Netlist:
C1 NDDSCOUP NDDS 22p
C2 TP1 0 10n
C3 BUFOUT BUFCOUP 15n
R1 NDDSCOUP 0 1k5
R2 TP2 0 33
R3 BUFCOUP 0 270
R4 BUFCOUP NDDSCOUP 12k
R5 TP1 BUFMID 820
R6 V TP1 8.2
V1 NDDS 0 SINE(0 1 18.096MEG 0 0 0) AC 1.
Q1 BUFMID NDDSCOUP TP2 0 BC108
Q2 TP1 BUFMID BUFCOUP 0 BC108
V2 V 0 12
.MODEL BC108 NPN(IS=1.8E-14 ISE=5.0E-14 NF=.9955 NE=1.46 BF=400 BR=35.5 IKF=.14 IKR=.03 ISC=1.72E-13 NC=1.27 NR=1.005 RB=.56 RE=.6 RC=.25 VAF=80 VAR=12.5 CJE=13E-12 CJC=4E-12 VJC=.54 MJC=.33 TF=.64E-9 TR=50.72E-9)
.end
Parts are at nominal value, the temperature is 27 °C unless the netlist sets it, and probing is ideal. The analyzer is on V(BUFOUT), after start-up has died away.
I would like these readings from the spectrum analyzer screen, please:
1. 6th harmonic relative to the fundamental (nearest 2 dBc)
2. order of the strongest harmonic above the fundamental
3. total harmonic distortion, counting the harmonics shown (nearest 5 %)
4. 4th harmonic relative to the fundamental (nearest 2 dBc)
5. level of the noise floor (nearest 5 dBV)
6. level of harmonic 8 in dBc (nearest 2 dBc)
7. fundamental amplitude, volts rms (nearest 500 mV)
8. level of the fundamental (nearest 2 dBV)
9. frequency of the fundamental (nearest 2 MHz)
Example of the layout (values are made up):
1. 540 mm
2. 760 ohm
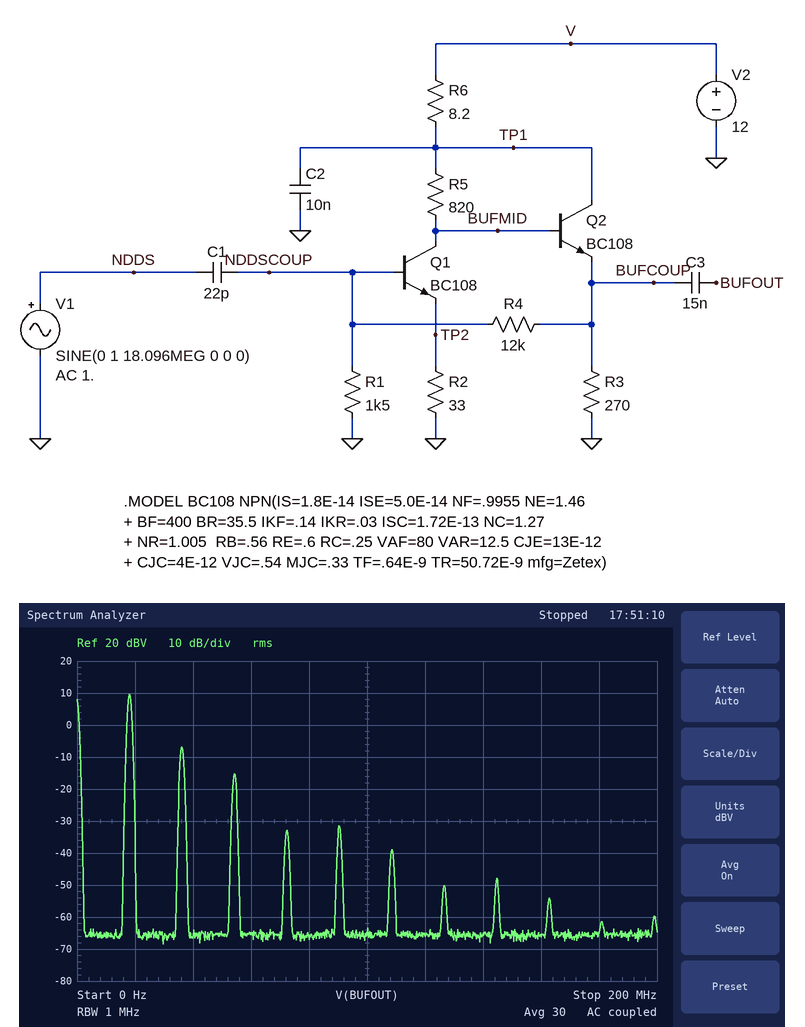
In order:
1. -48 dBc
2. 2
3. 15 %
4. -42 dBc
5. -65 dBV
6. -58 dBc
7. 3.0 V
8. 10 dBV
9. 18 MHz
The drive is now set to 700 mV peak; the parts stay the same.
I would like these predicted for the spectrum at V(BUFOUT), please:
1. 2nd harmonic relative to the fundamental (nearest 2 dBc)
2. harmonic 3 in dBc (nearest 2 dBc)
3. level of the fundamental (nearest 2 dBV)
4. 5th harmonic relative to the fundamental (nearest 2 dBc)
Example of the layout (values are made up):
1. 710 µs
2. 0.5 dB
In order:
1. -22 dBc
2. -30 dBc
3. 8 dBV
4. -58 dBc
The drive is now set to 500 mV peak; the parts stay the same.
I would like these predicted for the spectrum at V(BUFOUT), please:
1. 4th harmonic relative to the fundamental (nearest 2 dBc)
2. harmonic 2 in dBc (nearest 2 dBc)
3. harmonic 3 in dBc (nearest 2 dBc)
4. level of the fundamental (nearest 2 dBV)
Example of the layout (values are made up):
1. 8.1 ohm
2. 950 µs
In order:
1. -52 dBc
2. -30 dBc
3. -38 dBc
4. 6 dBV
